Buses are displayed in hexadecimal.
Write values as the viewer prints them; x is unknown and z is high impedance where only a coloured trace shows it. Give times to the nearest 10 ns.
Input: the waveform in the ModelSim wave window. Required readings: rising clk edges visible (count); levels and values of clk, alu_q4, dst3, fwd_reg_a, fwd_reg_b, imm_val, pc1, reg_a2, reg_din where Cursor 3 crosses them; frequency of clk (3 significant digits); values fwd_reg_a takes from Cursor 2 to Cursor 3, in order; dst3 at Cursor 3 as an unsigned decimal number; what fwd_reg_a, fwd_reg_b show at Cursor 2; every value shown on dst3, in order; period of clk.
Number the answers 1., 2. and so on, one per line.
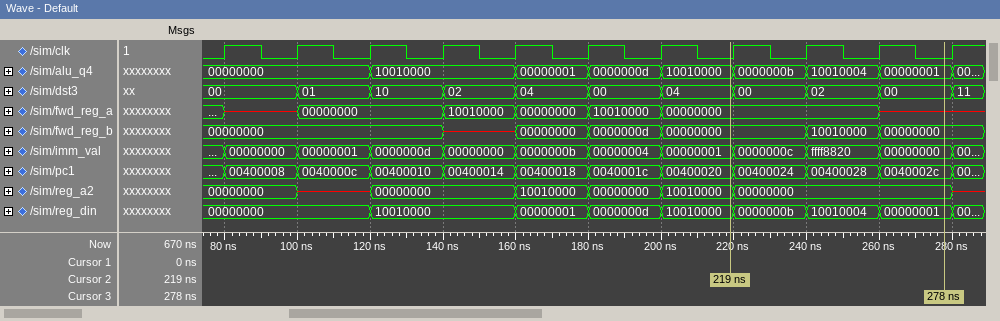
1. 11
2. clk=0, alu_q4=00000001, dst3=00, fwd_reg_a=x, fwd_reg_b=00000000, imm_val=00000000, pc1=0040002c, reg_a2=00000000, reg_din=00000001
3. 50.0 MHz
4. 00000000, x
5. 0
6. fwd_reg_a=00000000, fwd_reg_b=00000000
7. 00, 01, 10, 02, 04, 00, 04, 00, 02, 00, 11
8. 20 ns
